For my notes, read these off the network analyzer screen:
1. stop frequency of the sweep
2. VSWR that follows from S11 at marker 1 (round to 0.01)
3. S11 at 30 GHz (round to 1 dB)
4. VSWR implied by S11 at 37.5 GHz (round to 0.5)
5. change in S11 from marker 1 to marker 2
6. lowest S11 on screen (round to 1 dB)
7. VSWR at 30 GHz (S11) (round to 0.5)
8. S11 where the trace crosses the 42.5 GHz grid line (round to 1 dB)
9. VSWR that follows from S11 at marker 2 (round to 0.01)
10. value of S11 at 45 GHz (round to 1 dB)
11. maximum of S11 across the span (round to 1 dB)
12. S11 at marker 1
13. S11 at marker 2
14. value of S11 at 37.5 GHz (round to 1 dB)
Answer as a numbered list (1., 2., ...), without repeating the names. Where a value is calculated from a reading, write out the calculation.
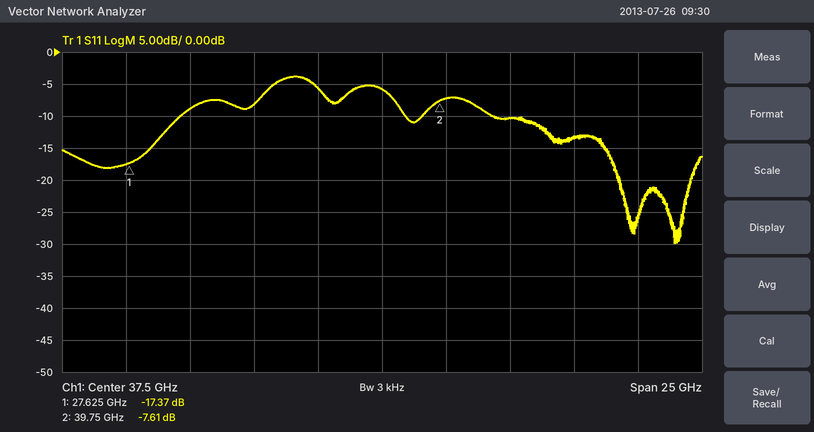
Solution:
1. 50 GHz
2. (1 + 0.1354)/(1 − 0.1354) ≈ 1.31
3. -9 dB
4. |Γ| = 10^(-6/20) = 0.5012; VSWR = (1 + 0.5012)/(1 − 0.5012) ≈ 3.0
5. -7.61 − (-17.37) = 9.76 dB
6. -30 dB
7. |Γ| = 10^(-9/20) = 0.3548; VSWR = (1 + 0.3548)/(1 − 0.3548) ≈ 2.10, so 2.0 to the nearest 0.5
8. -10 dB
9. (1 + 0.4164)/(1 − 0.4164) ≈ 2.43
10. -13 dB
11. -4 dB
12. -17.37 dB
13. -7.61 dB
14. -6 dB
